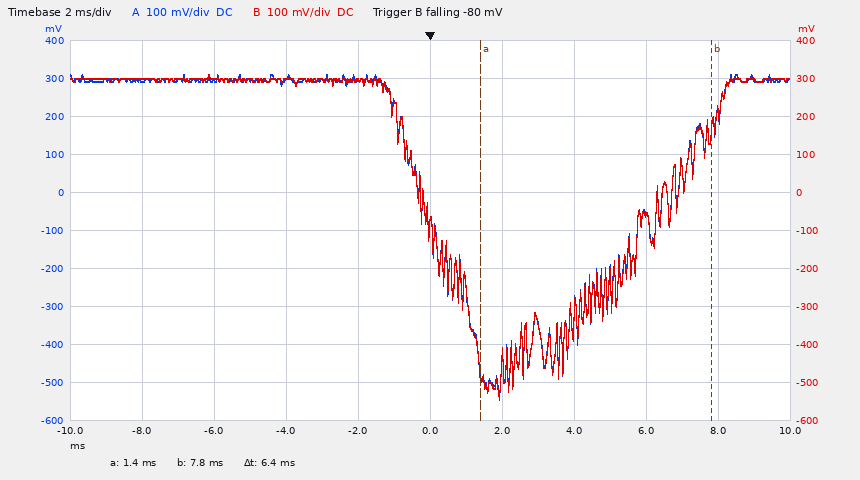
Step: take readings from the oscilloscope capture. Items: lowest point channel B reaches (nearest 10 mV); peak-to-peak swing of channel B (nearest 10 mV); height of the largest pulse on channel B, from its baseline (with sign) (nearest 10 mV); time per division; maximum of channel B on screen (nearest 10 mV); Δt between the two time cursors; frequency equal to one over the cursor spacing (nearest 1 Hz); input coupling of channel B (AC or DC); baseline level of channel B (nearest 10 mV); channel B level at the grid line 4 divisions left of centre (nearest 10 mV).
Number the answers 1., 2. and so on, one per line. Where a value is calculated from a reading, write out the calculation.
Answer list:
1. -540 mV
2. 310 mV − (-540 mV) = 850 mV
3. -540 mV − (300 mV) = -840 mV
4. 2 ms
5. 310 mV
6. 6.4 ms
7. 1 / 6.4 ms ≈ 156 Hz
8. DC
9. 300 mV
10. 300 mV
